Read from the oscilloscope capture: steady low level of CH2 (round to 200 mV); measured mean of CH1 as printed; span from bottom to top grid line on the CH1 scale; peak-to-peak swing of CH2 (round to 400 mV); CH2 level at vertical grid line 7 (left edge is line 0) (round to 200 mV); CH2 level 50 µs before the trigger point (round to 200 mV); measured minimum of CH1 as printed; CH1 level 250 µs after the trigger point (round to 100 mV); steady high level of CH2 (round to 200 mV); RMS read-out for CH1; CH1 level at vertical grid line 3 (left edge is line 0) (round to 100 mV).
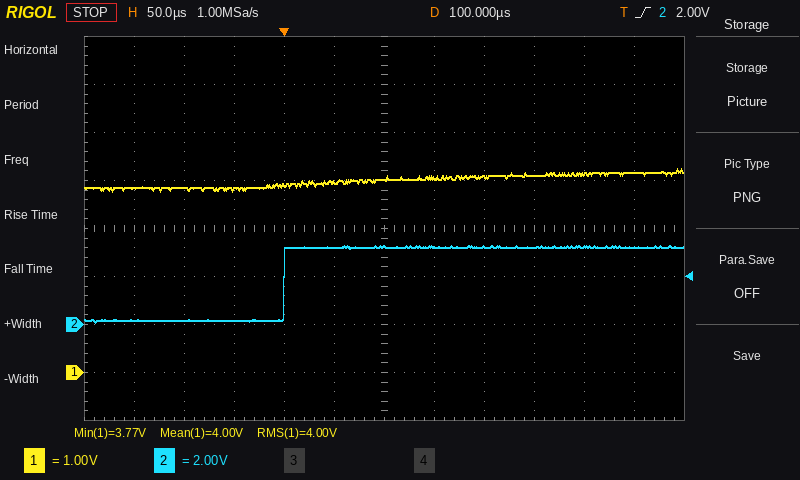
200 mV
4.00 V
8 V
3.2 V
3.2 V
200 mV
3.77 V
4.1 V
3.2 V
4.00 V
3.8 V
